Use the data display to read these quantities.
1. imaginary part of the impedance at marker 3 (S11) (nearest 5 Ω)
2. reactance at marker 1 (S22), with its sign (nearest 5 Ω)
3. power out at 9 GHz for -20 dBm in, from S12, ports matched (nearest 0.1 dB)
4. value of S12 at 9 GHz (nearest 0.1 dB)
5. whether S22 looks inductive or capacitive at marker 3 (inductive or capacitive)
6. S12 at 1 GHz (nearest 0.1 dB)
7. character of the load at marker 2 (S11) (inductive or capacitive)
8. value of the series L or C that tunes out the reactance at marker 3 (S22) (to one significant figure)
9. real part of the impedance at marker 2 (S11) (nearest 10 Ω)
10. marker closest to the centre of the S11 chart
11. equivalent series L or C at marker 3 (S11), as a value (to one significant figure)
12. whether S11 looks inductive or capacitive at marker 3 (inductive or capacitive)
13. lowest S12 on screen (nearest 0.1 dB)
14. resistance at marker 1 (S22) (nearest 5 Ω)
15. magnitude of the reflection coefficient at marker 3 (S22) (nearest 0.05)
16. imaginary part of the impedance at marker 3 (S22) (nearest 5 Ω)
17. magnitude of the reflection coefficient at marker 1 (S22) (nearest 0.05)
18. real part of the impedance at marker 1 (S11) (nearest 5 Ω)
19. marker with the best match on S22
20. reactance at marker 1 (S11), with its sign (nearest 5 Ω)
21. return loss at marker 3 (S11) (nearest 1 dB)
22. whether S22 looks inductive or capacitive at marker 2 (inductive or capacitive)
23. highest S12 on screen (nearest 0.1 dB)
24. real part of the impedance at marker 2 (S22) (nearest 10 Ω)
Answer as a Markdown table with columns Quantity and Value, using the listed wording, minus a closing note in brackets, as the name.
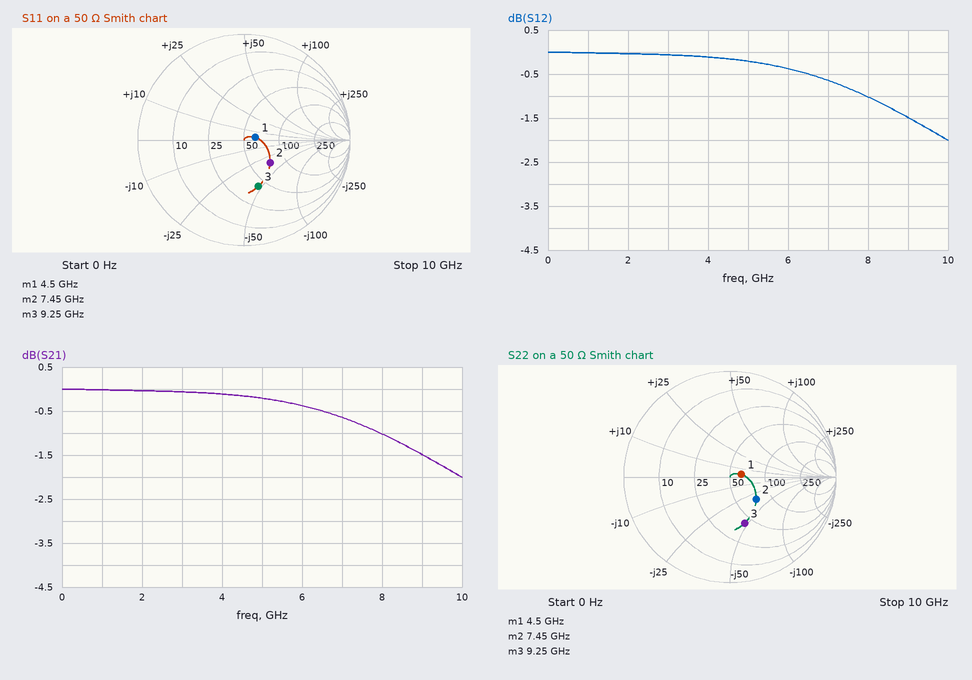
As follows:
| Quantity | Value |
|---|---|
| imaginary part of the impedance at marker 3 (S11) | -45 Ω |
| reactance at marker 1 (S22), with its sign | +5 Ω |
| power out at 9 GHz for -20 dBm in, from S12, ports matched | -21.5 dBm |
| value of S12 at 9 GHz | -1.5 dB |
| whether S22 looks inductive or capacitive at marker 3 | capacitive |
| S12 at 1 GHz | 0.0 dB |
| character of the load at marker 2 (S11) | capacitive |
| value of the series L or C that tunes out the reactance at marker 3 (S22) | 800 pH |
| real part of the impedance at marker 2 (S11) | 70 Ω |
| marker closest to the centre of the S11 chart | marker 1 |
| equivalent series L or C at marker 3 (S11), as a value | 400 fF |
| whether S11 looks inductive or capacitive at marker 3 | capacitive |
| lowest S12 on screen | -2.0 dB |
| resistance at marker 1 (S22) | 60 Ω |
| magnitude of the reflection coefficient at marker 3 (S22) | 0.45 |
| imaginary part of the impedance at marker 3 (S22) | -45 Ω |
| magnitude of the reflection coefficient at marker 1 (S22) | 0.10 |
| real part of the impedance at marker 1 (S11) | 60 Ω |
| marker with the best match on S22 | marker 1 |
| reactance at marker 1 (S11), with its sign | +5 Ω |
| return loss at marker 3 (S11) | 7 dB |
| whether S22 looks inductive or capacitive at marker 2 | capacitive |
| highest S12 on screen | 0.0 dB |
| real part of the impedance at marker 2 (S22) | 70 Ω |
